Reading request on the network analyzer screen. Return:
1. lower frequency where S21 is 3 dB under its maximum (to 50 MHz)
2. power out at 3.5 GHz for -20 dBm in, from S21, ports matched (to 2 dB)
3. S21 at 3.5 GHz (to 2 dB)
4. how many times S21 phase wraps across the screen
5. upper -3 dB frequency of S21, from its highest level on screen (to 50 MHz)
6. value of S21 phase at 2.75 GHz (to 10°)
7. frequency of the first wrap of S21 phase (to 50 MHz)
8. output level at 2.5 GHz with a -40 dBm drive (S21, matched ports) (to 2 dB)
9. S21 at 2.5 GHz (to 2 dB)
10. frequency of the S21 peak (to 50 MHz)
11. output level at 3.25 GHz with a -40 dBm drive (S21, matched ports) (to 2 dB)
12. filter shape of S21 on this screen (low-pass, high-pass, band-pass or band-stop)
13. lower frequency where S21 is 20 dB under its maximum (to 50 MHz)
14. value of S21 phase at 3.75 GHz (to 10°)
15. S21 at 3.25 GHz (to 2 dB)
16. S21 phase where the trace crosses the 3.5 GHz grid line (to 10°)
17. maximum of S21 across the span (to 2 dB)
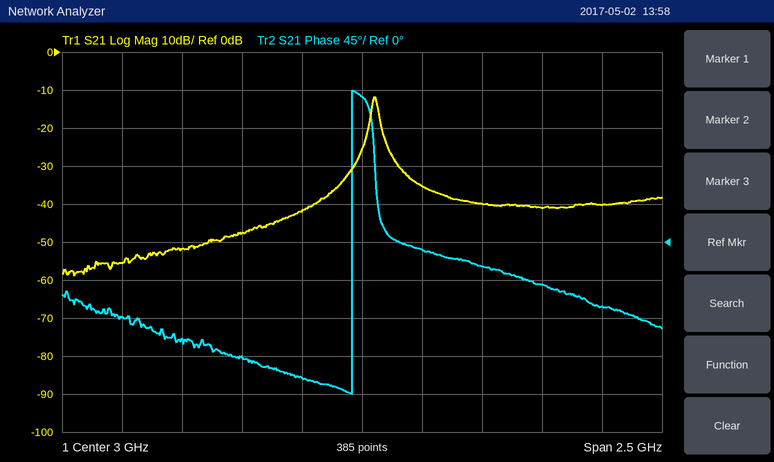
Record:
3.05 GHz
-60 dBm
-40 dB
1
3.05 GHz
-160°
2.95 GHz
-88 dBm
-48 dB
3.05 GHz
-76 dBm
band-pass
2.95 GHz
-50°
-36 dB
-30°
-12 dB
